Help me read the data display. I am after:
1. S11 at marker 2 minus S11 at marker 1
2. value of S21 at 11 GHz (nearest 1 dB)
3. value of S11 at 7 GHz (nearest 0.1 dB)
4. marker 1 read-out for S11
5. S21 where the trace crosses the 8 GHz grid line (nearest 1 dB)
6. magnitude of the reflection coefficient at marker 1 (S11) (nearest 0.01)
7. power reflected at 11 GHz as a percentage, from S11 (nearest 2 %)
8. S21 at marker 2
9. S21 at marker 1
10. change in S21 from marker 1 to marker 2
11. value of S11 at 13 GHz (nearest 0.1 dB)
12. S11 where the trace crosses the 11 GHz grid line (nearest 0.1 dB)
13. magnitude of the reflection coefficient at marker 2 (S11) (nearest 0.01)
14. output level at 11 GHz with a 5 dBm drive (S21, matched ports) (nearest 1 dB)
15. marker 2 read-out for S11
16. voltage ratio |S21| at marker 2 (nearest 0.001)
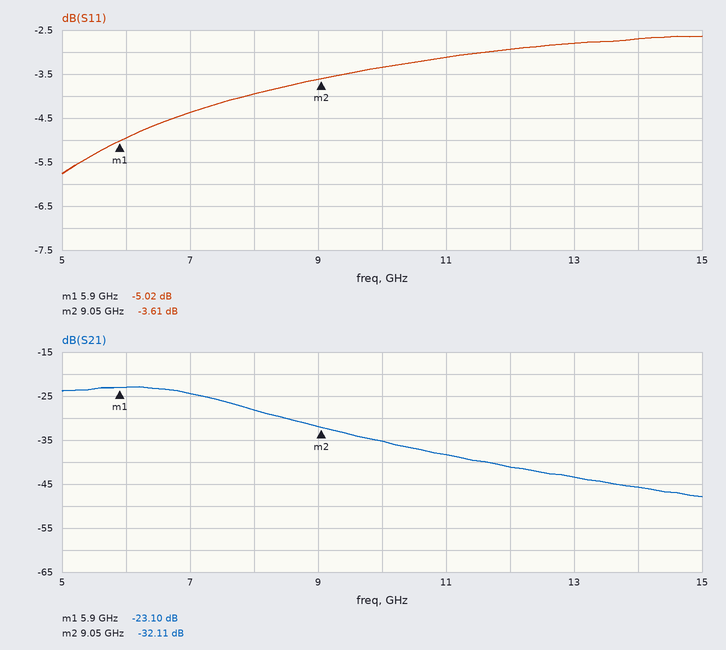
1.41 dB
-38 dB
-4.4 dB
-5.02 dB
-28 dB
0.56
48 %
-32.11 dB
-23.10 dB
-9.01 dB
-2.8 dB
-3.1 dB
0.66
-33 dBm
-3.61 dB
0.025
